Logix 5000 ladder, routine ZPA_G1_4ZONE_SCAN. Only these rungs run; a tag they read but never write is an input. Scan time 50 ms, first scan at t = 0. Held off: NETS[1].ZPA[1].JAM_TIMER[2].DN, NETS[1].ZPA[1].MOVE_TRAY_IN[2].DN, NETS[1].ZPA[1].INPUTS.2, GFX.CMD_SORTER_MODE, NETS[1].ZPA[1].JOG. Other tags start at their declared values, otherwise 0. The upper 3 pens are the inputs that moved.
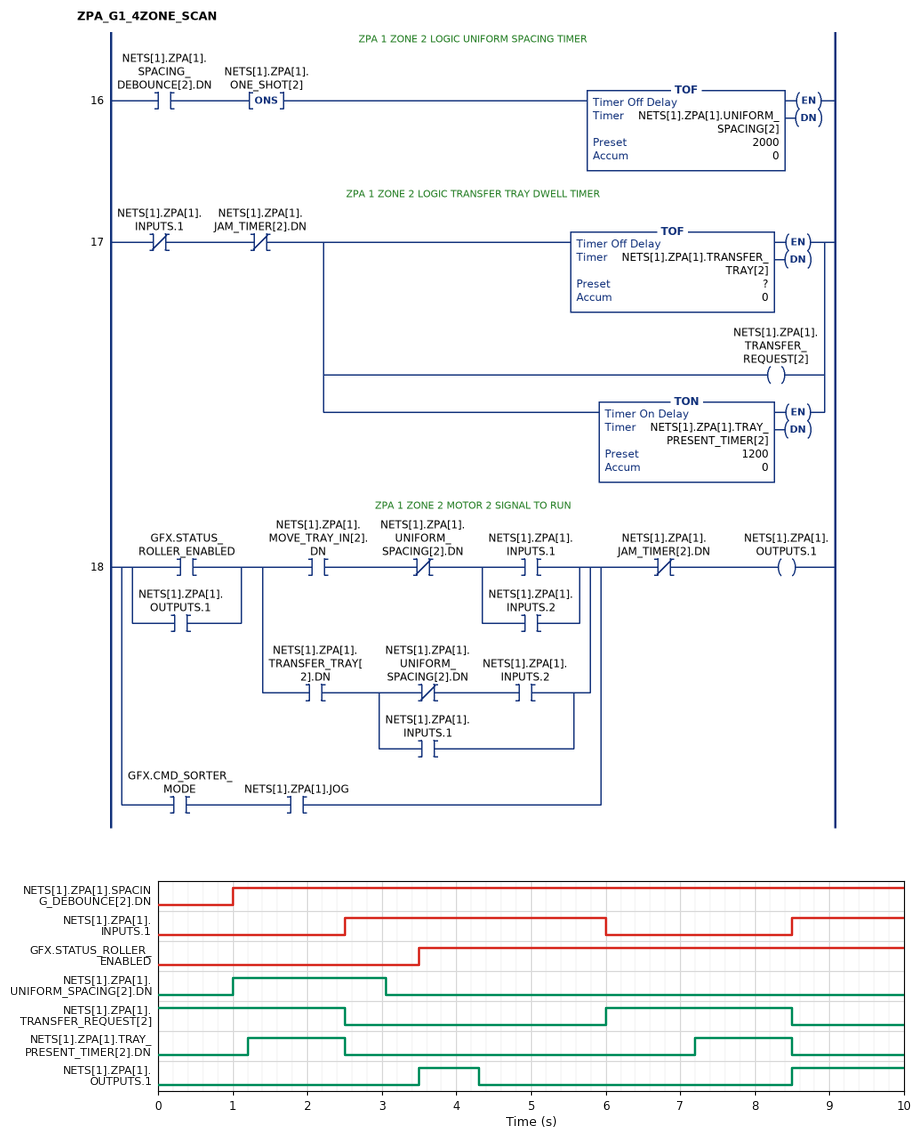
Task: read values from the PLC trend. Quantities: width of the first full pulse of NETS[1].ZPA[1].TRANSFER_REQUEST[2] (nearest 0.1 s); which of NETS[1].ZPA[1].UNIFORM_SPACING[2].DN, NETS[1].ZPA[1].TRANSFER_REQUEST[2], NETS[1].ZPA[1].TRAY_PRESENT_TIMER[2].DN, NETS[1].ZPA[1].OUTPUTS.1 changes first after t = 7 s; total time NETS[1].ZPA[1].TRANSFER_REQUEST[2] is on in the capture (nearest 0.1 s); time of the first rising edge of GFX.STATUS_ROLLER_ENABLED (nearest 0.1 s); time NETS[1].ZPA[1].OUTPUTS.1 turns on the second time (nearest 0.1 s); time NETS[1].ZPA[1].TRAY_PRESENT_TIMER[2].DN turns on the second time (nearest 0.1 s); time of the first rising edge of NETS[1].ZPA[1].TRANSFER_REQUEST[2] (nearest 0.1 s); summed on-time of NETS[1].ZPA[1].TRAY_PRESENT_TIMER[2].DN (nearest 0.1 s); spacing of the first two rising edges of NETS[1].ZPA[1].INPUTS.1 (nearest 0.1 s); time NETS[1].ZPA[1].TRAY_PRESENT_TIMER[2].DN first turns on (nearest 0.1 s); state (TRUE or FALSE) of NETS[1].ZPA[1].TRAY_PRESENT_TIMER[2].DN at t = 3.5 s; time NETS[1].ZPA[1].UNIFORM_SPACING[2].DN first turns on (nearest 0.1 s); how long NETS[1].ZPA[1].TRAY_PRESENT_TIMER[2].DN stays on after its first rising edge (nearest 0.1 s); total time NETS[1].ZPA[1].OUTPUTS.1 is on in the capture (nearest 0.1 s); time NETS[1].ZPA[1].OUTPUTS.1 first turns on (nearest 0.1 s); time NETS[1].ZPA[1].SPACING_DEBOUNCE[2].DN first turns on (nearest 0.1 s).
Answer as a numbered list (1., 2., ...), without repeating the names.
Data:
1. 2.5 s
2. NETS[1].ZPA[1].TRAY_PRESENT_TIMER[2].DN
3. 5.0 s
4. 3.5 s
5. 8.5 s
6. 7.2 s
7. 6.0 s
8. 2.6 s
9. 6.0 s
10. 1.2 s
11. FALSE
12. 1.0 s
13. 1.3 s
14. 2.3 s
15. 3.5 s
16. 1.0 s
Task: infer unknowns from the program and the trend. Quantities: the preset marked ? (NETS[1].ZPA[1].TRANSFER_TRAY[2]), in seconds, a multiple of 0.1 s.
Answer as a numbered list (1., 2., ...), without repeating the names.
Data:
1. 1.8 s
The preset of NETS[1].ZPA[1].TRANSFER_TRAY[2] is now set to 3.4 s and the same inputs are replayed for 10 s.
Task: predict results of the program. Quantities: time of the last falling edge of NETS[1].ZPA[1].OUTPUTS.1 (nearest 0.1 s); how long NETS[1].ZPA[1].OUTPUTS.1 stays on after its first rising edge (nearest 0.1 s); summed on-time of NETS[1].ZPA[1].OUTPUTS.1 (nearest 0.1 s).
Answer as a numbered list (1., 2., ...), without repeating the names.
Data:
1. 5.9 s
2. 2.4 s
3. 3.9 s
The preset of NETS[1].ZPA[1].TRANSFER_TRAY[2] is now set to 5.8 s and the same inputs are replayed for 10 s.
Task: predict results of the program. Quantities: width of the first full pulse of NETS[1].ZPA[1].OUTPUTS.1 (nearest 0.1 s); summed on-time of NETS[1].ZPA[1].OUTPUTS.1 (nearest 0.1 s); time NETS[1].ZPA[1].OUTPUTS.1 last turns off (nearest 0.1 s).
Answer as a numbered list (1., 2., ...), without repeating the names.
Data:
1. 2.5 s
2. 4.0 s
3. 6.0 s
